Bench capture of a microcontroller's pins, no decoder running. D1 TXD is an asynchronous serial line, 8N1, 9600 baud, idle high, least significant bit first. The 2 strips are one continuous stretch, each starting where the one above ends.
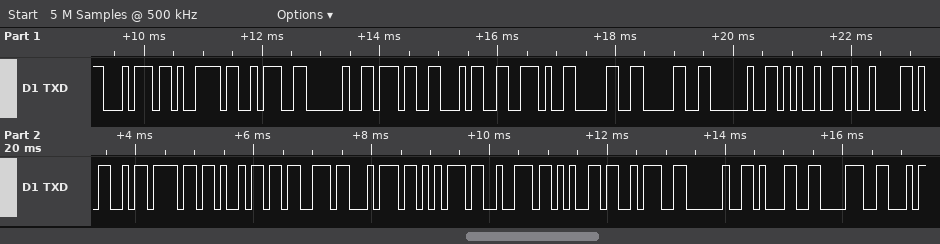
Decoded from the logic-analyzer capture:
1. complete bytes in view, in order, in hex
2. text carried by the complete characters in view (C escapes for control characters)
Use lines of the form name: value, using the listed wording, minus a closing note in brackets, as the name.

complete bytes in view, in order, in hex: 0x74 0x79 0x3A 0x20 0x37 0x34 0x2E 0x30 0x30 0x20 0x25 0x09 0x4D 0x6F 0x69 0x73 0x74 0x75 0x72 0x65 0x3A 0x20 0x31 0x38
text carried by the complete characters in view: "ty: 74.00 %\tMoisture: 18"
